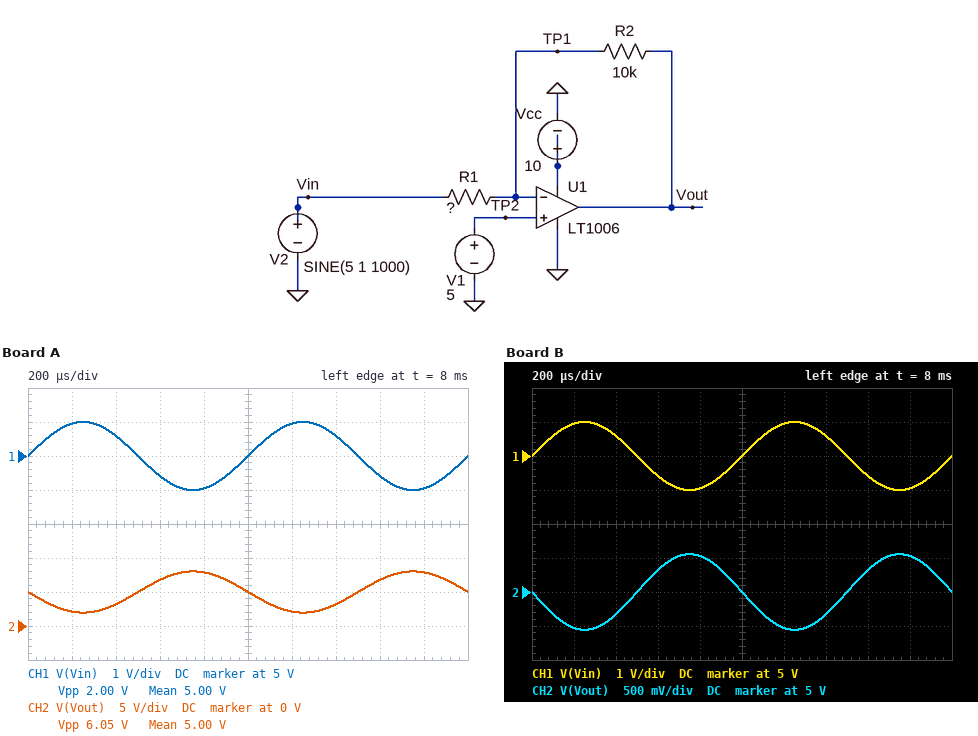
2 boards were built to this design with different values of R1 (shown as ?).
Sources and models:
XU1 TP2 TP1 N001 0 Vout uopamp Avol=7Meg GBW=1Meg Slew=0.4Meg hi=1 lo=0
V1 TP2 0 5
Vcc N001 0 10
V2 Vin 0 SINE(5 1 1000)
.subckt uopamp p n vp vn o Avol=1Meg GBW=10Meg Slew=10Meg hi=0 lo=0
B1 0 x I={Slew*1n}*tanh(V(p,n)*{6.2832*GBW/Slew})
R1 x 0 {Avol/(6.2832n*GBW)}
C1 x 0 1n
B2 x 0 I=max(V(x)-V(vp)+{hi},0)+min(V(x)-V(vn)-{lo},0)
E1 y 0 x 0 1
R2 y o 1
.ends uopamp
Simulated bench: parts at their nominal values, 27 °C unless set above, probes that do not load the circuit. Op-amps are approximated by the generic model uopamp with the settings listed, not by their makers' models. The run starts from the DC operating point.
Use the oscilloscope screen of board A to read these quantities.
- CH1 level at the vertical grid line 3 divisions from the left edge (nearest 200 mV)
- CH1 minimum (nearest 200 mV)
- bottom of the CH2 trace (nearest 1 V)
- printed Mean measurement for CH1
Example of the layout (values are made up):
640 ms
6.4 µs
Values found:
4.4 V
4.0 V
2 V
5.00 V
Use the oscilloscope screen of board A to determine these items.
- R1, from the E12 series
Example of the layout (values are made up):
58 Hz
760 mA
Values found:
3.3 kΩ
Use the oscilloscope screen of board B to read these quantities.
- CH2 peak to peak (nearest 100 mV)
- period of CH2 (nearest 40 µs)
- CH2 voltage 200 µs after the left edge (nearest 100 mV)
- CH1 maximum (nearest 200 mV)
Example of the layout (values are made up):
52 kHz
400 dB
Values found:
1.1 V
1.00 ms
4.5 V
6.0 V
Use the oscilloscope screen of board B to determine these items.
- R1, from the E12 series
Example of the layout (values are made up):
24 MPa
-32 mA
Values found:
18 kΩ
